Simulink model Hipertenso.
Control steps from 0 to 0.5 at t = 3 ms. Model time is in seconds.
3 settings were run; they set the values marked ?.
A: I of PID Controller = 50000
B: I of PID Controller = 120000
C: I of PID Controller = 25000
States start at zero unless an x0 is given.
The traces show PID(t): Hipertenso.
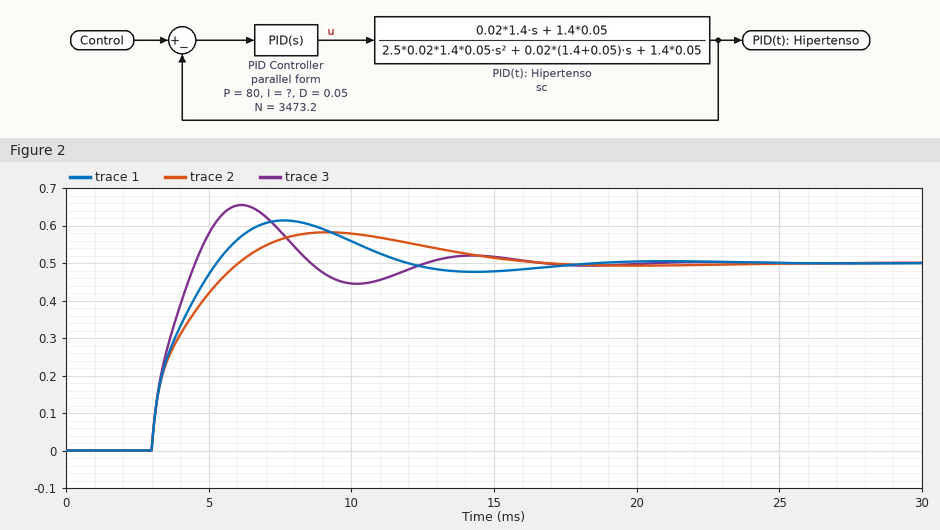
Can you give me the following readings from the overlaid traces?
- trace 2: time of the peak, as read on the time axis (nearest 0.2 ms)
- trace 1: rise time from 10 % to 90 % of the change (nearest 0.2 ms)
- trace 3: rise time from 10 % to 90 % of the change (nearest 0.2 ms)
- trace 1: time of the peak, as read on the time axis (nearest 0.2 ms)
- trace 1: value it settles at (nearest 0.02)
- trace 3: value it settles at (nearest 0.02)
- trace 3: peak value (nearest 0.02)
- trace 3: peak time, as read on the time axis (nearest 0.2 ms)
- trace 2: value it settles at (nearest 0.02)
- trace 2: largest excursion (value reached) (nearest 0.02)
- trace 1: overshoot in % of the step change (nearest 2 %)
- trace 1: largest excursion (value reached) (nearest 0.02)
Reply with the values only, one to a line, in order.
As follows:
9.2 ms
1.8 ms
1.2 ms
7.6 ms
0.50
0.50
0.66
6.2 ms
0.50
0.58
22 %
0.62
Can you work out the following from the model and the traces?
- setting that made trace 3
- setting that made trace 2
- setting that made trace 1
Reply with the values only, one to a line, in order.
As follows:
B
C
A
